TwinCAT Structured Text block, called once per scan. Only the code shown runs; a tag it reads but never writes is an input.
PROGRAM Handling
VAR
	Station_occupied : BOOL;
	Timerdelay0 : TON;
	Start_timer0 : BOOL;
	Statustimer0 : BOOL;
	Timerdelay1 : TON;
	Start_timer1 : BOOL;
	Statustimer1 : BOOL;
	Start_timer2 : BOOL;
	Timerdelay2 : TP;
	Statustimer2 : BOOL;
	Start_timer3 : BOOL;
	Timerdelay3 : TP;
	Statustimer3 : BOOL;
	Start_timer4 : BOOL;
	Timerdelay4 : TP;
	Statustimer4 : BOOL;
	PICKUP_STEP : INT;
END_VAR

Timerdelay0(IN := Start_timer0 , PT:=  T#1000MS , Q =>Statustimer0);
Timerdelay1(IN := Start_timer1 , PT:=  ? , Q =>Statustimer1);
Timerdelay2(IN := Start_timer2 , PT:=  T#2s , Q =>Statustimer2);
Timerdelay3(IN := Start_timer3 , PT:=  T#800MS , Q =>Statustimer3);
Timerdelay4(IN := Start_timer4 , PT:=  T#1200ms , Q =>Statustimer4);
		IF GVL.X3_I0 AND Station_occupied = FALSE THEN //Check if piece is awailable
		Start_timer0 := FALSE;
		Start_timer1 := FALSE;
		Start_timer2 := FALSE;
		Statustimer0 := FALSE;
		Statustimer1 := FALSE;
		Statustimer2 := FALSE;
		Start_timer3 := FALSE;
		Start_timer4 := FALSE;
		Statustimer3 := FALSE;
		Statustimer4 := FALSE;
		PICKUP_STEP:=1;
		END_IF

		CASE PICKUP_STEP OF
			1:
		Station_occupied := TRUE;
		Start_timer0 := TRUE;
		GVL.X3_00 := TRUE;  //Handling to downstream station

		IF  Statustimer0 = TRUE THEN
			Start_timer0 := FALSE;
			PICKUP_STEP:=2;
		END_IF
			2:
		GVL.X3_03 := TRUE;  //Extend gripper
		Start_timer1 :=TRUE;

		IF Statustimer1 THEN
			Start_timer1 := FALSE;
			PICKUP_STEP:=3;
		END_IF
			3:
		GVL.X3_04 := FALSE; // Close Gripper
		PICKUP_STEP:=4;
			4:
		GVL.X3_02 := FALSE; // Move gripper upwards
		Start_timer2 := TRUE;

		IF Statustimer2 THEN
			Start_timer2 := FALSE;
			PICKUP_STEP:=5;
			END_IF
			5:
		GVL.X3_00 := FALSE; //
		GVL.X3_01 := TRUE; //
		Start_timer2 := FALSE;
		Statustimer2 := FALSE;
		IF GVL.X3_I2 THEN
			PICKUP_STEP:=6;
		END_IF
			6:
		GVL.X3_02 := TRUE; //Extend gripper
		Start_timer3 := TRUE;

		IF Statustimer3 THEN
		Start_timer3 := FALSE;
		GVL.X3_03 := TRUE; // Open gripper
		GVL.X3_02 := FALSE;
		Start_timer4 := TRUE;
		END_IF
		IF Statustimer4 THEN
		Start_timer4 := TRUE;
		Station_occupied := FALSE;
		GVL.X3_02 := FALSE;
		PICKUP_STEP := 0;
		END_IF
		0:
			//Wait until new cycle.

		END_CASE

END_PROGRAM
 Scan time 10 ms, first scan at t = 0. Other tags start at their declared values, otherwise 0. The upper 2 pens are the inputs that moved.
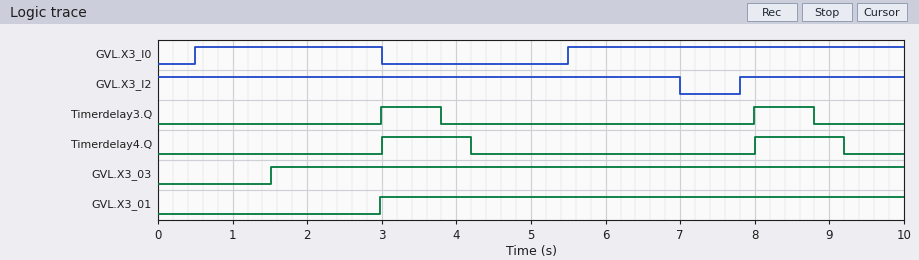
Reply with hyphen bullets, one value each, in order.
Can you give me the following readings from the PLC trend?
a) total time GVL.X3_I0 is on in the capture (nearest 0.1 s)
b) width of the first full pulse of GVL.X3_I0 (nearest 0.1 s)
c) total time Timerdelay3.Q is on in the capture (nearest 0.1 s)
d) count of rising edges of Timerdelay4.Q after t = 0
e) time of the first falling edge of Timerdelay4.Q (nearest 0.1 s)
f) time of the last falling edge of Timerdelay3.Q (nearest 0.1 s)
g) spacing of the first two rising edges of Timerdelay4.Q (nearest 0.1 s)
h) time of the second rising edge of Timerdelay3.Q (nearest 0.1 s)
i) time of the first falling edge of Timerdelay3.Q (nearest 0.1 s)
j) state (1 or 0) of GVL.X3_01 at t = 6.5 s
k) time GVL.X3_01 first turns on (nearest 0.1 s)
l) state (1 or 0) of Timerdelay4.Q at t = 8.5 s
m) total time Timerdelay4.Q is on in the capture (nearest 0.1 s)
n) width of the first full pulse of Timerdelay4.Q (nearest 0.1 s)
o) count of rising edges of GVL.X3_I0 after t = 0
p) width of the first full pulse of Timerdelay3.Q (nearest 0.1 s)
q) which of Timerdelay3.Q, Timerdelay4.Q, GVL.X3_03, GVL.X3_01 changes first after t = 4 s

- 7.0 s
- 2.5 s
- 1.6 s
- 2
- 4.2 s
- 8.8 s
- 5.0 s
- 8.0 s
- 3.8 s
- 1
- 3.0 s
- 1
- 2.4 s
- 1.2 s
- 2
- 0.8 s
- Timerdelay4.Q
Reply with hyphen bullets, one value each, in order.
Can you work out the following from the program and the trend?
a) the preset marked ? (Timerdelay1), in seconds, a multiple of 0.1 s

- 1.4 s
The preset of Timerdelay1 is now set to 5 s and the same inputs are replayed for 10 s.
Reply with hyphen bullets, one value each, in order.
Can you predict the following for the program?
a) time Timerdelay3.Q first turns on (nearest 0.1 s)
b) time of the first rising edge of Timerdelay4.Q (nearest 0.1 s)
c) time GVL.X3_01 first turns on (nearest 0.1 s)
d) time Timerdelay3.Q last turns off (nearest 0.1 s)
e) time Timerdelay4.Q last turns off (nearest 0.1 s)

- 6.6 s
- 6.6 s
- 6.6 s
- 7.4 s
- 7.8 s
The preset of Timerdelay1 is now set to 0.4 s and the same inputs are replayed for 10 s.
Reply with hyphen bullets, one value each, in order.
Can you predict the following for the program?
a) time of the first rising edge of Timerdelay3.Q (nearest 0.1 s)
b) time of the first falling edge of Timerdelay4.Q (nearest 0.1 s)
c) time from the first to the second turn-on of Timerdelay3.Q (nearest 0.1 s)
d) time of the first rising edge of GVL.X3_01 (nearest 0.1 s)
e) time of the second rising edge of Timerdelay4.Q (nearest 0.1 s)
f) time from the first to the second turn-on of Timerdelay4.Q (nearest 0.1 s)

- 2.0 s
- 3.2 s
- 1.5 s
- 2.0 s
- 3.5 s
- 1.5 s
